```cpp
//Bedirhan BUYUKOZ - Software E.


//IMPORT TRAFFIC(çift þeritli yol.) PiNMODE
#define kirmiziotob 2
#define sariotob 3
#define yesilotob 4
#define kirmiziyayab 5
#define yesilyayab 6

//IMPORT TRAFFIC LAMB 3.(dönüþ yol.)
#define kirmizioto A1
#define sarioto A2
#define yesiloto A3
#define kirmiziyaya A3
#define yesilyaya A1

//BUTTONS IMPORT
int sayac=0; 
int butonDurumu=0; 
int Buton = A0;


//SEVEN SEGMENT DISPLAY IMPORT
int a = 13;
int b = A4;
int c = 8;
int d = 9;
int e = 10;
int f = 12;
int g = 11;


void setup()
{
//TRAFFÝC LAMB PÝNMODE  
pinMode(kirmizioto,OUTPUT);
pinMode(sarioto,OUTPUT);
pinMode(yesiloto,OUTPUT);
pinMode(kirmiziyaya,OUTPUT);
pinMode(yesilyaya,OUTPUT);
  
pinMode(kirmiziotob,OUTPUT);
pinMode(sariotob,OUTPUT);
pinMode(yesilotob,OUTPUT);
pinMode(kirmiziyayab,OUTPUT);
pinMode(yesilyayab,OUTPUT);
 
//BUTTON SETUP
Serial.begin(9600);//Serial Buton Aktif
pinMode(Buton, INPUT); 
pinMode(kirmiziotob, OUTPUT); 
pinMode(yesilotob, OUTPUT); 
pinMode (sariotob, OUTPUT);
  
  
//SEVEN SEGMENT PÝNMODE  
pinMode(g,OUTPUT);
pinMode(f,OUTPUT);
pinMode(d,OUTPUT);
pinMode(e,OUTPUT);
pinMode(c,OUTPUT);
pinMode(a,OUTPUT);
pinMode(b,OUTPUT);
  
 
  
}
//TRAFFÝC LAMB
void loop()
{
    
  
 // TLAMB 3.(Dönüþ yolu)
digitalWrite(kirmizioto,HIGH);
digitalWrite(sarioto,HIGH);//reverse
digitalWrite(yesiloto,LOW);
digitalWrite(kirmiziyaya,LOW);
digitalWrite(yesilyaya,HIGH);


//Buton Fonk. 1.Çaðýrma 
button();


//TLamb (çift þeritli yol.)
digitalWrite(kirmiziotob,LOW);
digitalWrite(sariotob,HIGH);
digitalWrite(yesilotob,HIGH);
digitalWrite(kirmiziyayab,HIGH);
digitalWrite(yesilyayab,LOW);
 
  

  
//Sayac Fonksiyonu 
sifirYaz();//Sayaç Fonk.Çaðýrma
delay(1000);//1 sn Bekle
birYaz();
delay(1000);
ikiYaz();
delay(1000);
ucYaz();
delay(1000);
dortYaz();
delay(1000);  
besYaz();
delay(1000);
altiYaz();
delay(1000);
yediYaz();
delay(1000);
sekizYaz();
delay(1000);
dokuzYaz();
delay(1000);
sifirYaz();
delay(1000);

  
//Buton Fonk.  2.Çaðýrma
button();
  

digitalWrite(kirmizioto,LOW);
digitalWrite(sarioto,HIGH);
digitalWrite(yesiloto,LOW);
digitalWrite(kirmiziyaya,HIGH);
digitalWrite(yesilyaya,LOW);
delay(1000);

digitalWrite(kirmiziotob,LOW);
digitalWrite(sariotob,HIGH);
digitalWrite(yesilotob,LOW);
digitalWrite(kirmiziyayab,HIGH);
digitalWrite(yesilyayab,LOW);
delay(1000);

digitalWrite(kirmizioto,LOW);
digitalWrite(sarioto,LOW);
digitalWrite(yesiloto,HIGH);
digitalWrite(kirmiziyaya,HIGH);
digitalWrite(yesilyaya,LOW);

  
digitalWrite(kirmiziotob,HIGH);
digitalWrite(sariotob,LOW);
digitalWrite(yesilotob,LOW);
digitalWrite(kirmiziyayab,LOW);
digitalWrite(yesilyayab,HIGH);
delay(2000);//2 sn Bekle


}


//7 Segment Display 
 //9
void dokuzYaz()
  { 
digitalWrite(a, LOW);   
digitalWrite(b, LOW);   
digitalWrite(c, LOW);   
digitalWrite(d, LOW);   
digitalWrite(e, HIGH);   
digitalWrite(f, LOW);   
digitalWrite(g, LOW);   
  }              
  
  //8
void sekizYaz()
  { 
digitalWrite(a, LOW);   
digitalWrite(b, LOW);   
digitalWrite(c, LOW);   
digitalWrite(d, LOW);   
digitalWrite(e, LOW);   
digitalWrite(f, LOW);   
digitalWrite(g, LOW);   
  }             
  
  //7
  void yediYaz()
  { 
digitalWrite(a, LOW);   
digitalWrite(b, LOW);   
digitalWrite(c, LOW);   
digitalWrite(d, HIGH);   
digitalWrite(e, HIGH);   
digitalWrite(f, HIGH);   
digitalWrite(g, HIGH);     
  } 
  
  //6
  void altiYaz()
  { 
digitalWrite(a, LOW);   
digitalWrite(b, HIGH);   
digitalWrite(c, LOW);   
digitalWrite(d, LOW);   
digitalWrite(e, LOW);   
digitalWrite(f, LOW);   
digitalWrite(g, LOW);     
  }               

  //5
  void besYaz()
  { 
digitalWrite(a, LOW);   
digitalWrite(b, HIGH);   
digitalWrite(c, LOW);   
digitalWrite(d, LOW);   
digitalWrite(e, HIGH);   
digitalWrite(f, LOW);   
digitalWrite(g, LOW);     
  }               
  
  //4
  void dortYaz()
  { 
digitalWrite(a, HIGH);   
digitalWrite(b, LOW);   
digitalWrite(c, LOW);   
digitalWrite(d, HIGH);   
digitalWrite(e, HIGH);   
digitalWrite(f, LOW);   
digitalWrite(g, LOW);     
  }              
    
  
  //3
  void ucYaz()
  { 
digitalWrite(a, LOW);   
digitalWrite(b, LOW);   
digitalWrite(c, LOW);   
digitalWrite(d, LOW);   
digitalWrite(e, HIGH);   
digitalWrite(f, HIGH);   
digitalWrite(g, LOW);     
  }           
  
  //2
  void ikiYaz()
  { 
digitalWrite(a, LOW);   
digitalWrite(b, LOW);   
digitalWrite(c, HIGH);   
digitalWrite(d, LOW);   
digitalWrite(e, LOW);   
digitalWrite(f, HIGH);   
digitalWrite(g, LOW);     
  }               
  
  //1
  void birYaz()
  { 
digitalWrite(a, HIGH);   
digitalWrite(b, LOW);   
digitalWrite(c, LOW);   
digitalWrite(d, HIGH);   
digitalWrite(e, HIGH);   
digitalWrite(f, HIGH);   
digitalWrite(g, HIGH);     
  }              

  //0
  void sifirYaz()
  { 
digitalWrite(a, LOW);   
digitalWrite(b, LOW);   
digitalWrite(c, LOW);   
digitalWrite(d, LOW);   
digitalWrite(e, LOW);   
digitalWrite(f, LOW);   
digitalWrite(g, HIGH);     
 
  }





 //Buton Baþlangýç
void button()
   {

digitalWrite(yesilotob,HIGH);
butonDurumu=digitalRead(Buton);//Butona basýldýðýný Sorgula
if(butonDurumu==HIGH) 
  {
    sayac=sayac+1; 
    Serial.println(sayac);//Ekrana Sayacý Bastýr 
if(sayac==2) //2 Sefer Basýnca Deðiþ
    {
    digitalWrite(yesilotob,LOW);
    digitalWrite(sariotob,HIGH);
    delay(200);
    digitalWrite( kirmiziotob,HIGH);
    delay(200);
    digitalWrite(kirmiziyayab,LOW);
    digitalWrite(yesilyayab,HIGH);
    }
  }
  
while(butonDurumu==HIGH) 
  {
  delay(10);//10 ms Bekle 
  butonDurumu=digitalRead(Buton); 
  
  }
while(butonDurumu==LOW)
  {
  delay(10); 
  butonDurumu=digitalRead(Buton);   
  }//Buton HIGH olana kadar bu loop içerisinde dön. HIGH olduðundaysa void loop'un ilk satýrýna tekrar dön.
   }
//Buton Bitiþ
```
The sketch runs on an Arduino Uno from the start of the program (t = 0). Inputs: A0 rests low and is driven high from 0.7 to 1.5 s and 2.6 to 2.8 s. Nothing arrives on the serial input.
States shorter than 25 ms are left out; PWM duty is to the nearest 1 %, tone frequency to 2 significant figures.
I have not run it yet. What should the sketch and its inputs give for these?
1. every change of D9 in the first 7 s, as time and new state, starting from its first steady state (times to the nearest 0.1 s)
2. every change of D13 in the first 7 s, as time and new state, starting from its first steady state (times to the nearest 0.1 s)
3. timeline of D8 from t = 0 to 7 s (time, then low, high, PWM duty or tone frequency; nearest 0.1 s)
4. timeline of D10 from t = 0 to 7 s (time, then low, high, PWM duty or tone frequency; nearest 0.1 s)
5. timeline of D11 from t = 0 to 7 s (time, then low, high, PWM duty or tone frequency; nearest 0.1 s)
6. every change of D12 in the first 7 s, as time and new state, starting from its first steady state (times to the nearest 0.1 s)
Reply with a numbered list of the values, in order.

1. 0 s low; 1.7 s high; 2.7 s low; 4.7 s high; 5.7 s low
2. 0 s low; 1.7 s high; 2.7 s low; 4.7 s high; 5.7 s low
3. 0 s low; 2.7 s high; 3.7 s low
4. 0 s low; 1.7 s high; 2.7 s low; 3.7 s high; 6.7 s low
5. 0 s low; 0.7 s high; 2.7 s low
6. 0 s low; 1.7 s high; 4.7 s low
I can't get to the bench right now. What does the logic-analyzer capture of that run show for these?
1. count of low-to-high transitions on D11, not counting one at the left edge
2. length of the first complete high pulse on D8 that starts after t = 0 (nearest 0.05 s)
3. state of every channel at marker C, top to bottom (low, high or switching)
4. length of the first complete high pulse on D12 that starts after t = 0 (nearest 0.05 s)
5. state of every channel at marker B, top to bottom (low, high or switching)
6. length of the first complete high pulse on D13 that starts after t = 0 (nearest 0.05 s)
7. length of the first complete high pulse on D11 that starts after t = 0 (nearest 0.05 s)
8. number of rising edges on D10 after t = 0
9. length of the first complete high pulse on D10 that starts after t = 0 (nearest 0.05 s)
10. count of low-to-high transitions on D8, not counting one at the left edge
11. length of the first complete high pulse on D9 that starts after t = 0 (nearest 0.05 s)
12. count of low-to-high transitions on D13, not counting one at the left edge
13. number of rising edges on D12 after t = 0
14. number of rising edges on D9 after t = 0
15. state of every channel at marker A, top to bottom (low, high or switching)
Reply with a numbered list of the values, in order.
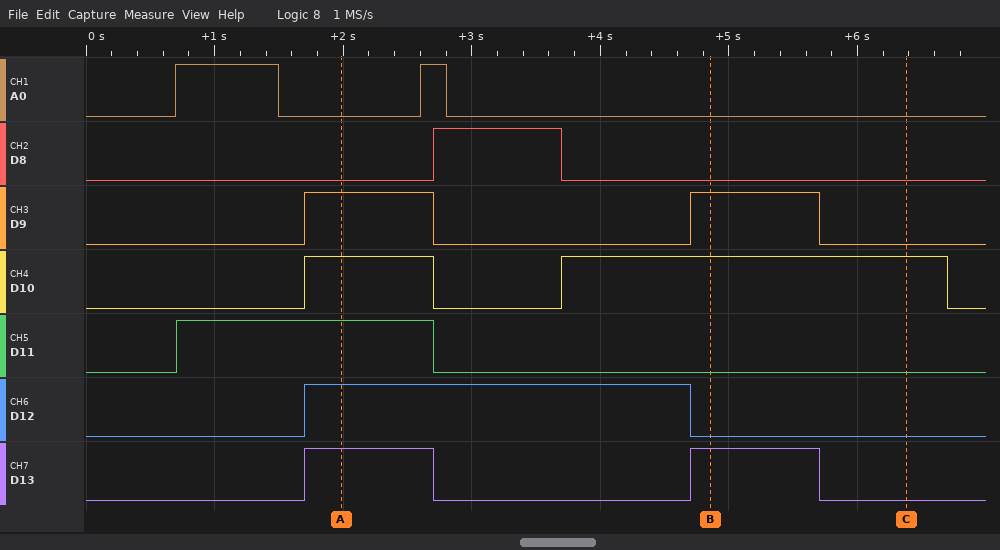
1. 1
2. 1.00 s
3. A0 low, D8 low, D9 low, D10 high, D11 low, D12 low, D13 low
4. 3.00 s
5. A0 low, D8 low, D9 high, D10 high, D11 low, D12 low, D13 high
6. 1.00 s
7. 2.00 s
8. 2
9. 1.00 s
10. 1
11. 1.00 s
12. 2
13. 1
14. 2
15. A0 low, D8 low, D9 high, D10 high, D11 high, D12 high, D13 high
